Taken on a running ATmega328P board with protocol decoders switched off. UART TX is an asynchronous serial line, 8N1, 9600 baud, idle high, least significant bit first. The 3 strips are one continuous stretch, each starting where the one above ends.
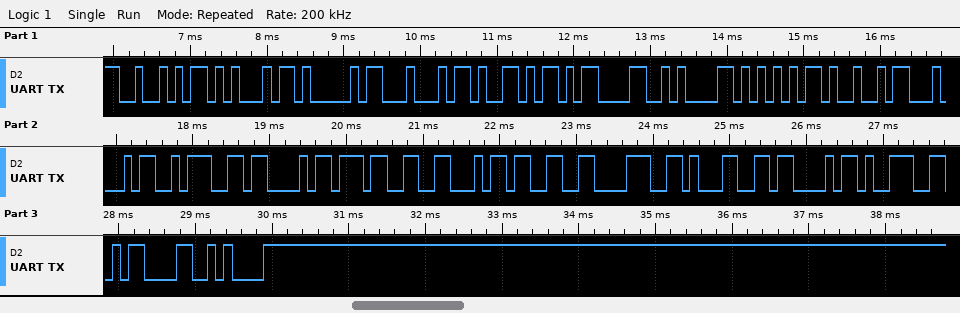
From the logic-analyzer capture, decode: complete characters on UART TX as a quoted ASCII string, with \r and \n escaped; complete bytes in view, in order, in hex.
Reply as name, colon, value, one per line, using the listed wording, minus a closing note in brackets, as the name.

complete characters on UART TX as a quoted ASCII string, with \r and \n escaped: "READY\r\nUID:C7F381C9\r\n"
complete bytes in view, in order, in hex: 52 45 41 44 59 0D 0A 55 49 44 3A 43 37 46 33 38 31 43 39 0D 0A
